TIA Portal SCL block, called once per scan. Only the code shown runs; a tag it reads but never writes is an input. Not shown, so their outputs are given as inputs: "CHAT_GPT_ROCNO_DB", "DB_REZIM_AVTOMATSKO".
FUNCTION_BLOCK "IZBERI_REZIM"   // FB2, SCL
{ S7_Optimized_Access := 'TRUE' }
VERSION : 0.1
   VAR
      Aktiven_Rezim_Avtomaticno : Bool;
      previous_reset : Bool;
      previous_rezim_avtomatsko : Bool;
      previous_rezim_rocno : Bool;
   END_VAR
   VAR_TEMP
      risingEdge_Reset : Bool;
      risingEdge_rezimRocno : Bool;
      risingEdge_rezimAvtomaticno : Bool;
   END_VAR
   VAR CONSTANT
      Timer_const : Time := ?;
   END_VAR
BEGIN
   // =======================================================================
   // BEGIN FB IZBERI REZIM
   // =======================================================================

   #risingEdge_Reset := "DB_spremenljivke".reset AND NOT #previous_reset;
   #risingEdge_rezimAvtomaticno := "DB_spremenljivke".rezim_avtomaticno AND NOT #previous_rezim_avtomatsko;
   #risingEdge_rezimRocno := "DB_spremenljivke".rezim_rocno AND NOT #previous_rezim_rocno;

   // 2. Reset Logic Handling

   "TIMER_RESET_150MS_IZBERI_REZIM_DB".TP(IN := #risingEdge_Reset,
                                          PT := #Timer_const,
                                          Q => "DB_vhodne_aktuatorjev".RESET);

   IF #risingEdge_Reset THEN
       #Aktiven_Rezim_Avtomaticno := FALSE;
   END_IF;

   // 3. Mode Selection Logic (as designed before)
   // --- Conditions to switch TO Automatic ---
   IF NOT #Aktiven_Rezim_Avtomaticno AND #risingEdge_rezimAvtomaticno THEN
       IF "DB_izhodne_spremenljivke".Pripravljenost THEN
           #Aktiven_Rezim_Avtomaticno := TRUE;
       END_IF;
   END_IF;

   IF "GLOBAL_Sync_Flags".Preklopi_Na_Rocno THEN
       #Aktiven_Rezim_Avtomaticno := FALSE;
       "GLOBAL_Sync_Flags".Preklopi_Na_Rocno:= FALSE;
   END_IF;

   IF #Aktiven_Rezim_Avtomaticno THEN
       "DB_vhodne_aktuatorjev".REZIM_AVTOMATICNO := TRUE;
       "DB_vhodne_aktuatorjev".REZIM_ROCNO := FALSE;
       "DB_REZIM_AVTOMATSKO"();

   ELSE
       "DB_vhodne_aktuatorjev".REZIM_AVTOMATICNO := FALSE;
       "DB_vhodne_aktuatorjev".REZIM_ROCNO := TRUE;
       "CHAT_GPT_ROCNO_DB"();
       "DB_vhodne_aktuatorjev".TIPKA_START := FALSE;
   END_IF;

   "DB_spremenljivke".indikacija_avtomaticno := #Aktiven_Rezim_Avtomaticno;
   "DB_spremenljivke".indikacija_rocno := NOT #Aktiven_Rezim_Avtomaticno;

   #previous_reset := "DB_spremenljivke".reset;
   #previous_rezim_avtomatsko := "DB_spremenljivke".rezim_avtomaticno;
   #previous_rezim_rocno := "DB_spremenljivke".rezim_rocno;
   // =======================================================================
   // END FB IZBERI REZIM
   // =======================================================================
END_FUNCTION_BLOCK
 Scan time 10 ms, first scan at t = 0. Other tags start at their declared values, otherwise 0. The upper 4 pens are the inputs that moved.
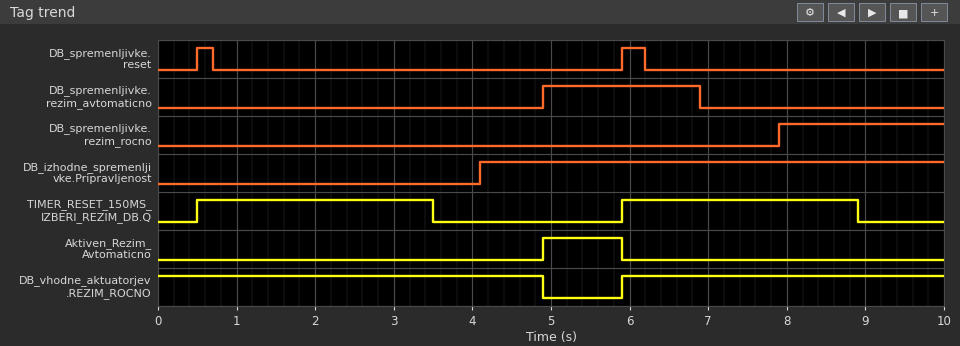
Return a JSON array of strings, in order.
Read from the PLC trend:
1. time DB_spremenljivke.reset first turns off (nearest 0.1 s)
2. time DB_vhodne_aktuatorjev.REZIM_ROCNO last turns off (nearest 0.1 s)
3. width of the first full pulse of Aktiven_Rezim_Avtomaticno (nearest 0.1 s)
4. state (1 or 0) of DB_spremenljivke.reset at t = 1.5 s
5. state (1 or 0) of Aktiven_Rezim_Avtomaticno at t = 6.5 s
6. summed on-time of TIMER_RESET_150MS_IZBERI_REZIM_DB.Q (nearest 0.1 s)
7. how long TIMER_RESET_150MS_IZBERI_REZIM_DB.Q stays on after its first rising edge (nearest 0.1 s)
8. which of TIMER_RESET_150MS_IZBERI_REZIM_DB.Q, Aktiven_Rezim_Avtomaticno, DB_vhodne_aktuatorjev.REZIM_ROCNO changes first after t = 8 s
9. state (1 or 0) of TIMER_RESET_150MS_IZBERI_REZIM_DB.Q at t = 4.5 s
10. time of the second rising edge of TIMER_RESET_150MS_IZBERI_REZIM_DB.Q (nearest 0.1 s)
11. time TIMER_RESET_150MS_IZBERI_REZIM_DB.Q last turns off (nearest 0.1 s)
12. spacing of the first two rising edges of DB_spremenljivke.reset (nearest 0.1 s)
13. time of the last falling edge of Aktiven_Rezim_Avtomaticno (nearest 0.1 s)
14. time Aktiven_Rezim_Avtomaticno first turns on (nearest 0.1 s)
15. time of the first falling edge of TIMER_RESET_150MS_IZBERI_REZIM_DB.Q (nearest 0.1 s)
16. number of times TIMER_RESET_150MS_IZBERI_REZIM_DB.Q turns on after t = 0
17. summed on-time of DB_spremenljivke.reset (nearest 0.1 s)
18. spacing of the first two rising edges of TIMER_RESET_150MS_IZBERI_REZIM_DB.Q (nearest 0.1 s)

["0.7 s", "4.9 s", "1.0 s", "0", "0", "6.0 s", "3.0 s", "TIMER_RESET_150MS_IZBERI_REZIM_DB.Q", "0", "5.9 s", "8.9 s", "5.4 s", "5.9 s", "4.9 s", "3.5 s", "2", "0.5 s", "5.4 s"]
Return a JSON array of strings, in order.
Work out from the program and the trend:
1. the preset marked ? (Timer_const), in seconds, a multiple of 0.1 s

["3.0 s"]
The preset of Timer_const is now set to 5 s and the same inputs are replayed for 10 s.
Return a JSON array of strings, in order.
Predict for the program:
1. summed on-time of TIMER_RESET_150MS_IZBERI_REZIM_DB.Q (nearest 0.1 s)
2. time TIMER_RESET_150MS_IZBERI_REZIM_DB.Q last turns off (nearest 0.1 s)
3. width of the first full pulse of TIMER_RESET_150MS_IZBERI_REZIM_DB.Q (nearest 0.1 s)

["9.1 s", "5.5 s", "5.0 s"]
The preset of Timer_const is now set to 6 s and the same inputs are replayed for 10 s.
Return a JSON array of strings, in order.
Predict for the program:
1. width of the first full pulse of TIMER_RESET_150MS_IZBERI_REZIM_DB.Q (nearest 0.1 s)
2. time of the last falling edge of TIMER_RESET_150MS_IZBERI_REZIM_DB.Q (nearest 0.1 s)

["6.0 s", "6.5 s"]
